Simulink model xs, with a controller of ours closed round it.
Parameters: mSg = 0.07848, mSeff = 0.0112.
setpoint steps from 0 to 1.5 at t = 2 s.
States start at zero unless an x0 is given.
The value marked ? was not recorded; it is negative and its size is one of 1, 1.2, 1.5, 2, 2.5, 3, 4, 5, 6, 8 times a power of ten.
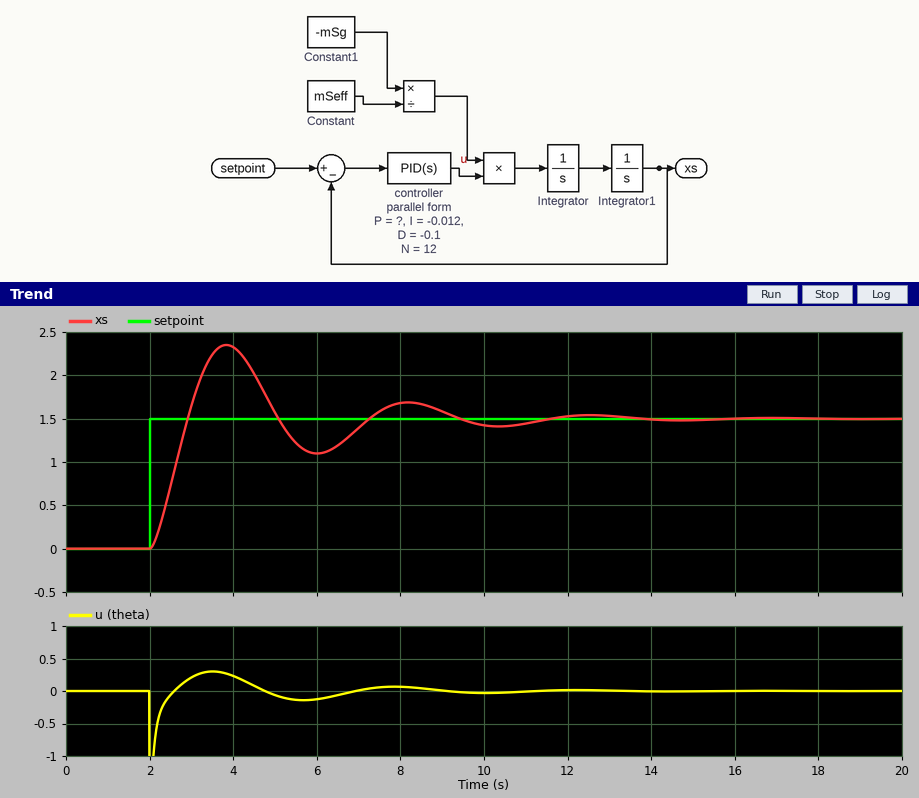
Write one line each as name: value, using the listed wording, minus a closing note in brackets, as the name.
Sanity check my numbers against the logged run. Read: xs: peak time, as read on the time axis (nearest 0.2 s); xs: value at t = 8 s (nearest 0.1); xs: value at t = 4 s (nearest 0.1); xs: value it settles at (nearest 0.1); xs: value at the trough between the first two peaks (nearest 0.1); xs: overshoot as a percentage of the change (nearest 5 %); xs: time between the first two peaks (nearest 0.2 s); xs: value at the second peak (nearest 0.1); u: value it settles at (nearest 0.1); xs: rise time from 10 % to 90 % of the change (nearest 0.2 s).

xs: peak time, as read on the time axis: 3.8 s
xs: value at t = 8 s: 1.7
xs: value at t = 4 s: 2.3
xs: value it settles at: 1.5
xs: value at the trough between the first two peaks: 1.1
xs: overshoot as a percentage of the change: 55 %
xs: time between the first two peaks: 4.4 s
xs: value at the second peak: 1.7
u: value it settles at: 0.0
xs: rise time from 10 % to 90 % of the change: 0.6 s
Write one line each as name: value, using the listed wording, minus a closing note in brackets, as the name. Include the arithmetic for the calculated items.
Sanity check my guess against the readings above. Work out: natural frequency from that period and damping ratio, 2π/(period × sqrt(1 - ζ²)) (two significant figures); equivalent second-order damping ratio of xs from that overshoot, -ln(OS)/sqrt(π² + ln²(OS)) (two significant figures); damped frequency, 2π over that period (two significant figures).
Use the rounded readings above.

natural frequency from that period and damping ratio, 2π/(period × sqrt(1 - ζ²)): 2π / (4.4 × sqrt(1 - 0.19²)) = 1.5 rad/s
equivalent second-order damping ratio of xs from that overshoot, -ln(OS)/sqrt(π² + ln²(OS)): ln(0.55) = -0.598; 0.598 / sqrt(9.870 + 0.357) = 0.19
damped frequency, 2π over that period: 2π / 4.4 = 1.4 rad/s
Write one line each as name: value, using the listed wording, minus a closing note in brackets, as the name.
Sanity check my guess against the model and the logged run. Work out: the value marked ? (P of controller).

the value marked ?: -0.3
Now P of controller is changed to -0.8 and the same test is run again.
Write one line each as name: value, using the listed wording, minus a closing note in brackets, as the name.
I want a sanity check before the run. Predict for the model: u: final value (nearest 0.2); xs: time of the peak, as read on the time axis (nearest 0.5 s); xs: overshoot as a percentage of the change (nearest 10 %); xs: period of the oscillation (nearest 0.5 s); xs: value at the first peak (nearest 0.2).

u: final value: 0.0
xs: time of the peak, as read on the time axis: 3.0 s
xs: overshoot as a percentage of the change: 70 %
xs: period of the oscillation: 2.5 s
xs: value at the first peak: 2.6
